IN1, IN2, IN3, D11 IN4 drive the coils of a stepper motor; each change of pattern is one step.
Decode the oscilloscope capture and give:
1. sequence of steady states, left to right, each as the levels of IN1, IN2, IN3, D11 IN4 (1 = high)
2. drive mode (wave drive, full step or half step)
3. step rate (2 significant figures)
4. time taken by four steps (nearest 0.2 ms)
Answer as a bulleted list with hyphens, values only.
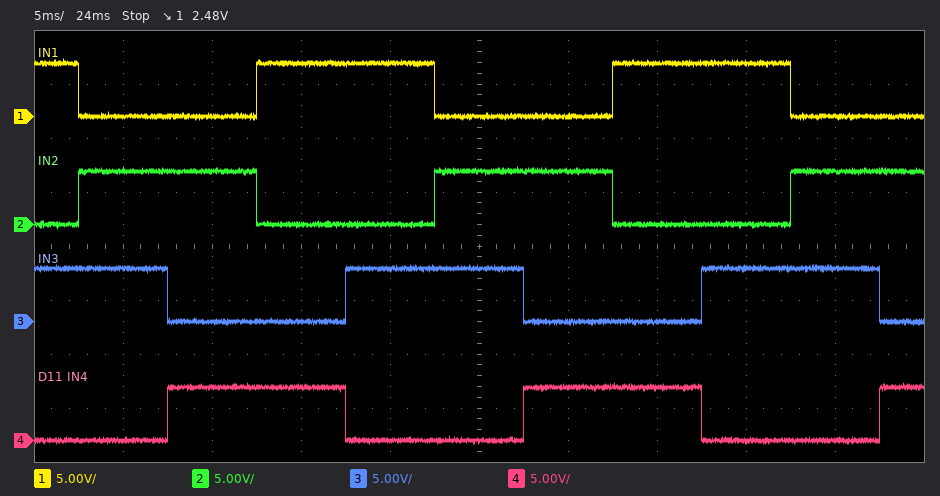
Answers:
- 1010 0110 0101 1001 1010 0110 0101 1001 1010 0110 0101
- full step
- 200 steps/s
- 20.0 ms
